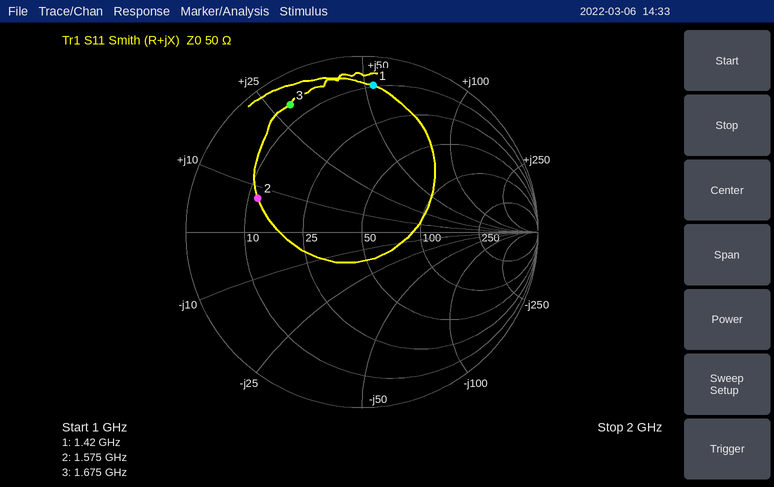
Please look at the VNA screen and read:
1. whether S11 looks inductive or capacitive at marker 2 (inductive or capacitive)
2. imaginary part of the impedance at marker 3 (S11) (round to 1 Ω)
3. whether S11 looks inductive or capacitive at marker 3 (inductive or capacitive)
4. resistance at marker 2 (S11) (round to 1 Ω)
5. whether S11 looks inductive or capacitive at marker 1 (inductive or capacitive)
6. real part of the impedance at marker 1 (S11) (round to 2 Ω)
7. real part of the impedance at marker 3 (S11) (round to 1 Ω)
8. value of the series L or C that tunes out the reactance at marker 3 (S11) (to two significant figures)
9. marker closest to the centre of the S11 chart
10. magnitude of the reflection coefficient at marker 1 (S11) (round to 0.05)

inductive
+29 Ω
inductive
12 Ω
inductive
10 Ω
6 Ω
3.3 pF
marker 2
0.85
